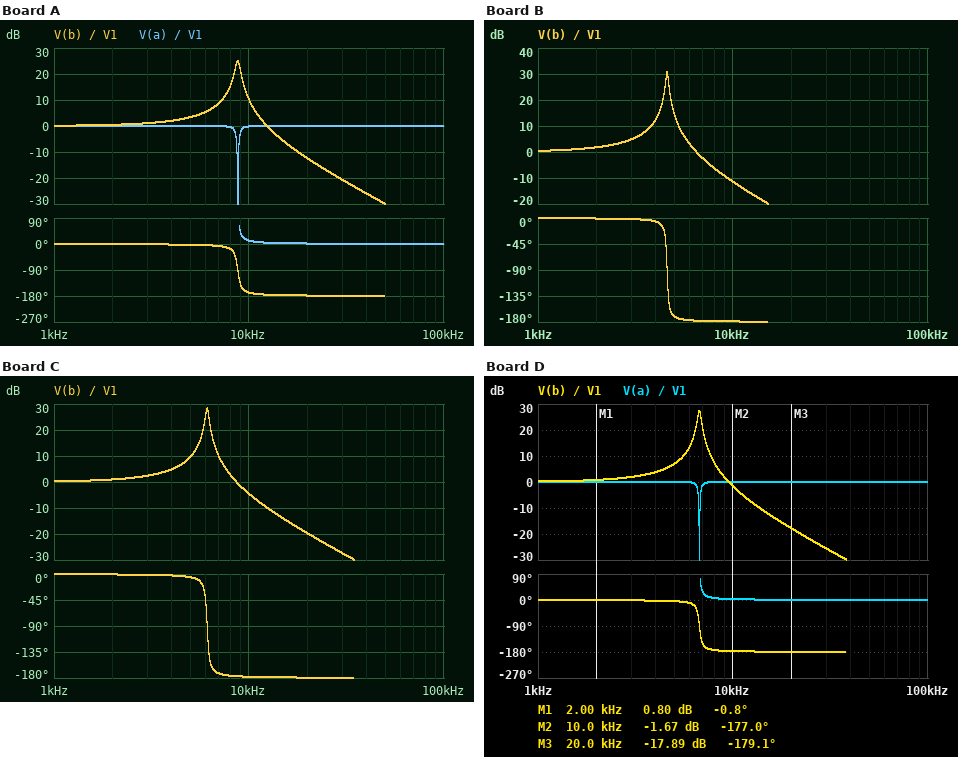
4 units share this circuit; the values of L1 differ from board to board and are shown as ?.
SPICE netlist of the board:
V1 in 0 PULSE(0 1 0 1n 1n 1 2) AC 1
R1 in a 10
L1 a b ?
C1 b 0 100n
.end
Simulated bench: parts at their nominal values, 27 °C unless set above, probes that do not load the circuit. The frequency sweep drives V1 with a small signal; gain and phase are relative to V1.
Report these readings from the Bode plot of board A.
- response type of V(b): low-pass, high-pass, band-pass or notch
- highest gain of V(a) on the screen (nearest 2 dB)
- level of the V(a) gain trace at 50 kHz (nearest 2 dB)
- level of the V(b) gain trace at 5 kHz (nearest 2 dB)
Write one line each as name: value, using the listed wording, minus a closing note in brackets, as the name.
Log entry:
response type of V(b): low-pass, high-pass, band-pass or notch: band-pass
highest gain of V(a) on the screen: 0 dB
level of the V(a) gain trace at 50 kHz: 0 dB
level of the V(b) gain trace at 5 kHz: 4 dB
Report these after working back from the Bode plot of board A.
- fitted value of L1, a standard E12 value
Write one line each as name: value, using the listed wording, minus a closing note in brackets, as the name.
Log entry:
fitted value of L1, a standard E12 value: 3.3 mH
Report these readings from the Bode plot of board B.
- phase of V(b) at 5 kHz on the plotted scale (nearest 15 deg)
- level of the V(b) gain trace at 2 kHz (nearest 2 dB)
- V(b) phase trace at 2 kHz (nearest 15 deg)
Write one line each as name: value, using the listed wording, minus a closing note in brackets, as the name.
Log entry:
phase of V(b) at 5 kHz on the plotted scale: -165 deg
level of the V(b) gain trace at 2 kHz: 2 dB
V(b) phase trace at 2 kHz: 0 deg
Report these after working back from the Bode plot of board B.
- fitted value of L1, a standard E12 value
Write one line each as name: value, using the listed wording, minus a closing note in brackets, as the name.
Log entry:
fitted value of L1, a standard E12 value: 12 mH
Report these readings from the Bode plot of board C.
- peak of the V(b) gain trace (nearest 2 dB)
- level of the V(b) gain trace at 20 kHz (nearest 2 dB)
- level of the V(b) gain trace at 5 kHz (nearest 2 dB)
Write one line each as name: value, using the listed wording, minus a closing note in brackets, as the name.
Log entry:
peak of the V(b) gain trace: 28 dB
level of the V(b) gain trace at 20 kHz: -20 dB
level of the V(b) gain trace at 5 kHz: 10 dB
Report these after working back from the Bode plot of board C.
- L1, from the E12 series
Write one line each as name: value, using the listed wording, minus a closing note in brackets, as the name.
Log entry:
L1, from the E12 series: 6.8 mH
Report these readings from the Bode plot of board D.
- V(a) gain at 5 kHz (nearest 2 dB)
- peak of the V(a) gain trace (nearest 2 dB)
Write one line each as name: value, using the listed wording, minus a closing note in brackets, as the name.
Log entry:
V(a) gain at 5 kHz: 0 dB
peak of the V(a) gain trace: 0 dB
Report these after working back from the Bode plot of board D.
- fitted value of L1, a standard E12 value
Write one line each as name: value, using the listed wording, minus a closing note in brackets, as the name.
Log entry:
fitted value of L1, a standard E12 value: 5.6 mH
